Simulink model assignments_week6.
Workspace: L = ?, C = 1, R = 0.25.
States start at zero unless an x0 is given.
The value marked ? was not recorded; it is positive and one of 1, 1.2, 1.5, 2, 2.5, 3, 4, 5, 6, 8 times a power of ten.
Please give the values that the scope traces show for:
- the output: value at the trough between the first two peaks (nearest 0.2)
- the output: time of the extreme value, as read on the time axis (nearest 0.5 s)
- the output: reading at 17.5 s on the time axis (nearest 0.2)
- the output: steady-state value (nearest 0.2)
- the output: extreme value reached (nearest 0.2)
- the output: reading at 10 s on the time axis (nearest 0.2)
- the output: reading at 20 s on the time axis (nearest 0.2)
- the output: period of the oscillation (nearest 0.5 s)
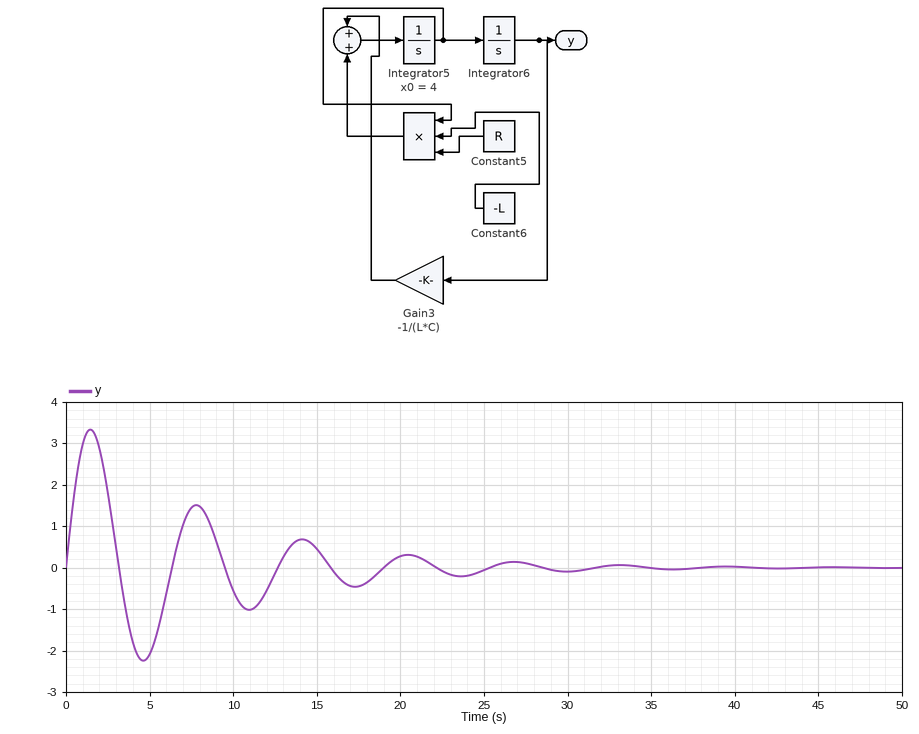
-2.2
1.5 s
-0.4
0.0
3.4
-0.6
0.2
6.5 s
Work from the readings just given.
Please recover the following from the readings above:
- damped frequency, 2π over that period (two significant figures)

0.97 rad/s
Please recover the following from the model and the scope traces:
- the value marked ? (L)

1
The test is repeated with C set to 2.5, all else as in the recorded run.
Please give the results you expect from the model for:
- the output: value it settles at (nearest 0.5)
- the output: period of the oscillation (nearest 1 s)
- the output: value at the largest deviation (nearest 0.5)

0.0
10 s
5.0
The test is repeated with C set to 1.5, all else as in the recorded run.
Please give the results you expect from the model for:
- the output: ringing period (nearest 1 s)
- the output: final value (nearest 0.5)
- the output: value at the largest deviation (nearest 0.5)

8 s
0.0
4.0
